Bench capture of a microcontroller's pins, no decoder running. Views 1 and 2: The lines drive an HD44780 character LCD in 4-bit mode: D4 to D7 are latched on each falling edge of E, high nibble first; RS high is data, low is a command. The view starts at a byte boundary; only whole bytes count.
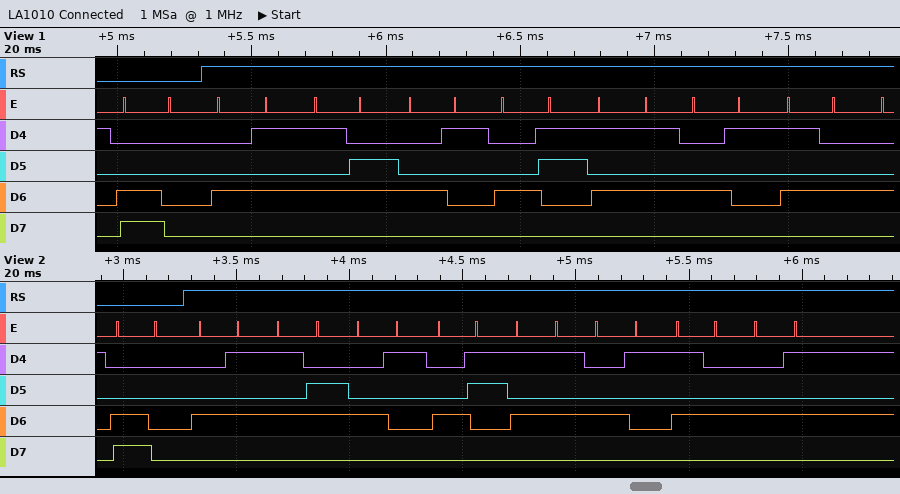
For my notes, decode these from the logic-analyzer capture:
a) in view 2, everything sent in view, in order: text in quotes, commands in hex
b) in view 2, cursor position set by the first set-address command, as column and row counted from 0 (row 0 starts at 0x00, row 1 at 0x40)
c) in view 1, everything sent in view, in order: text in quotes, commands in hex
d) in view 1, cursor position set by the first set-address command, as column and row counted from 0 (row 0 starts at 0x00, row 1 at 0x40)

0xC0 "EVACUATE"
column 0, row 1
0xC0 "EVACUAT"
column 0, row 1
